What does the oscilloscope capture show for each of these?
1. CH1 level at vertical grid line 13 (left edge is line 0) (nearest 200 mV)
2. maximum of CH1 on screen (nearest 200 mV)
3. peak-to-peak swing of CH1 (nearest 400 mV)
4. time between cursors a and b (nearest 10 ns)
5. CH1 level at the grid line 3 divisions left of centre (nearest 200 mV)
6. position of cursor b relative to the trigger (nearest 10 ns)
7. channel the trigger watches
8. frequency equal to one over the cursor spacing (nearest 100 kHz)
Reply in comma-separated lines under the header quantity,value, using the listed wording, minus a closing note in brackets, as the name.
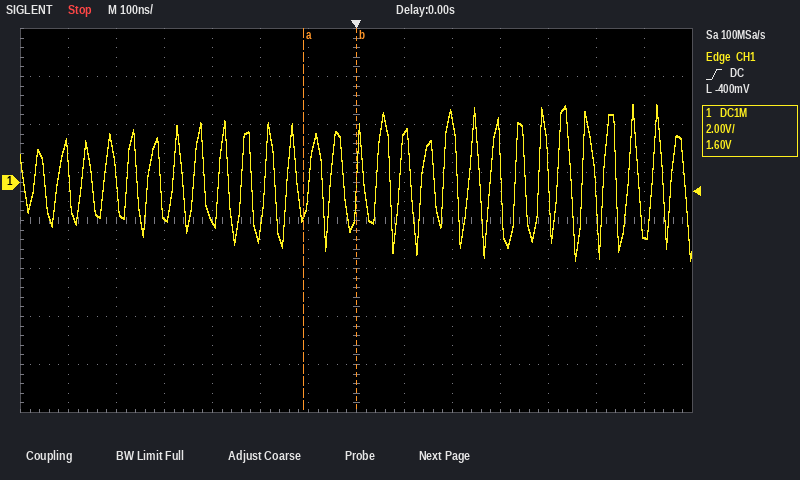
quantity,value
CH1 level at vertical grid line 13 (left edge is line 0),-2.2 V
maximum of CH1 on screen,3.2 V
peak-to-peak swing of CH1,6.4 V
time between cursors a and b,110 ns
CH1 level at the grid line 3 divisions left of centre,-1.6 V
position of cursor b relative to the trigger,0 ns
channel the trigger watches,CH1
frequency equal to one over the cursor spacing,9.1 MHz
